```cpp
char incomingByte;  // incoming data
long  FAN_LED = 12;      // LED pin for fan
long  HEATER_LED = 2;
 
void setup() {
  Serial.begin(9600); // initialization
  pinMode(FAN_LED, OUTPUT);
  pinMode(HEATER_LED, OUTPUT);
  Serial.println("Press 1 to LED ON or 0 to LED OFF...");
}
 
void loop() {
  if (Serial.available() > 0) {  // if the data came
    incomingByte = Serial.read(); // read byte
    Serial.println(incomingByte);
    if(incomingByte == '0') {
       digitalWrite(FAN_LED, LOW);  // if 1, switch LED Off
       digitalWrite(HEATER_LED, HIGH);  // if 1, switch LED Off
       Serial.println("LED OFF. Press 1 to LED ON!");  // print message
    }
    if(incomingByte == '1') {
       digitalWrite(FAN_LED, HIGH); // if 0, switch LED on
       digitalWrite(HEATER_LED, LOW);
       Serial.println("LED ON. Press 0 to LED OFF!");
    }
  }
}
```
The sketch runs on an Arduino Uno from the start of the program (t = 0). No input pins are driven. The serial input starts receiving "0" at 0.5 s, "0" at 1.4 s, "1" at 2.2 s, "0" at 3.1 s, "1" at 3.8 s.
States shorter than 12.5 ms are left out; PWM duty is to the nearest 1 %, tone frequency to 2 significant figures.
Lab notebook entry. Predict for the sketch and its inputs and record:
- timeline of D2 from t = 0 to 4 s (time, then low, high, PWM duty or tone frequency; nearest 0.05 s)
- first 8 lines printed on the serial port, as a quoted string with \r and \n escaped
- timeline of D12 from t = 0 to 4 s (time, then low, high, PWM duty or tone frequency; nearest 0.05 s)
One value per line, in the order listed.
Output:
0 s low; 0.5 s high; 2.2 s low; 3.1 s high; 3.8 s low
"Press 1 to LED ON or 0 to LED OFF...\r\n0\r\nLED OFF. Press 1 to LED ON!\r\n0\r\nLED OFF. Press 1 to LED ON!\r\n1\r\nLED ON. Press 0 to LED OFF!\r\n0\r\n"
0 s low; 2.2 s high; 3.1 s low; 3.8 s high
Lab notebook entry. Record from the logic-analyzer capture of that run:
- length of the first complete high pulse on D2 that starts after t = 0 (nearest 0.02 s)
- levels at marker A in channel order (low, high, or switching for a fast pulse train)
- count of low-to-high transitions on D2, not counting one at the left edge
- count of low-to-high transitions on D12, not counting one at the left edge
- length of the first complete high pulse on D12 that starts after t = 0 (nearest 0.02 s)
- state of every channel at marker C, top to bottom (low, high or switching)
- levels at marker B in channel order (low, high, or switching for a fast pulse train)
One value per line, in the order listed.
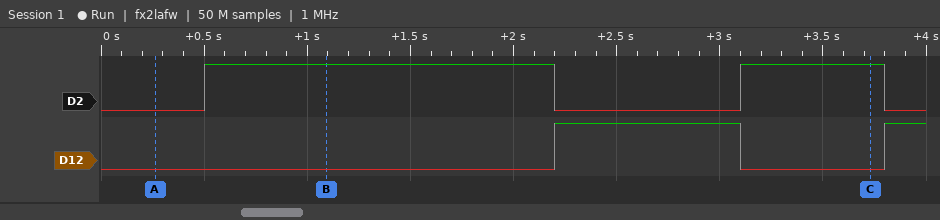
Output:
1.70 s
D2 low, D12 low
2
2
0.90 s
D2 high, D12 low
D2 high, D12 low
